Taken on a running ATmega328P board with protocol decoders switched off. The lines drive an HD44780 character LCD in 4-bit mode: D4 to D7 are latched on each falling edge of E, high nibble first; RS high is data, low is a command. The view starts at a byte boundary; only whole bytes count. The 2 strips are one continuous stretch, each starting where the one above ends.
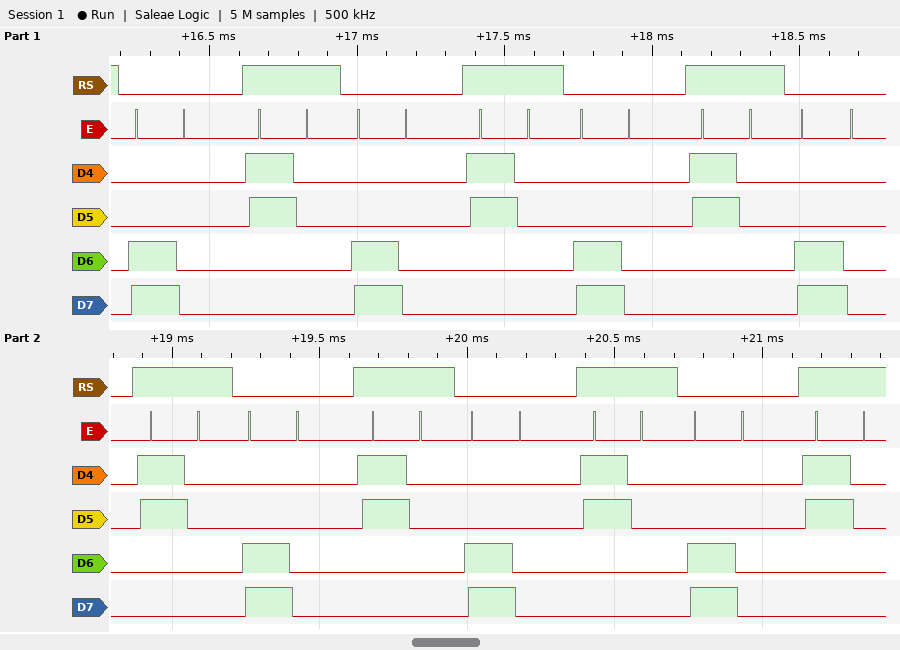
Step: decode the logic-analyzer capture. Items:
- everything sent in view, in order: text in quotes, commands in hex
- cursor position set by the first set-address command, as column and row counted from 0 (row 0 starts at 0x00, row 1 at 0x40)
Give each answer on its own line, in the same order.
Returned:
0xC0 "0" 0xC0 "0" 0xC0 "0" 0xC0 "0" 0xC0 "0" 0xC0 "0" 0xC0 "0"
column 0, row 1
